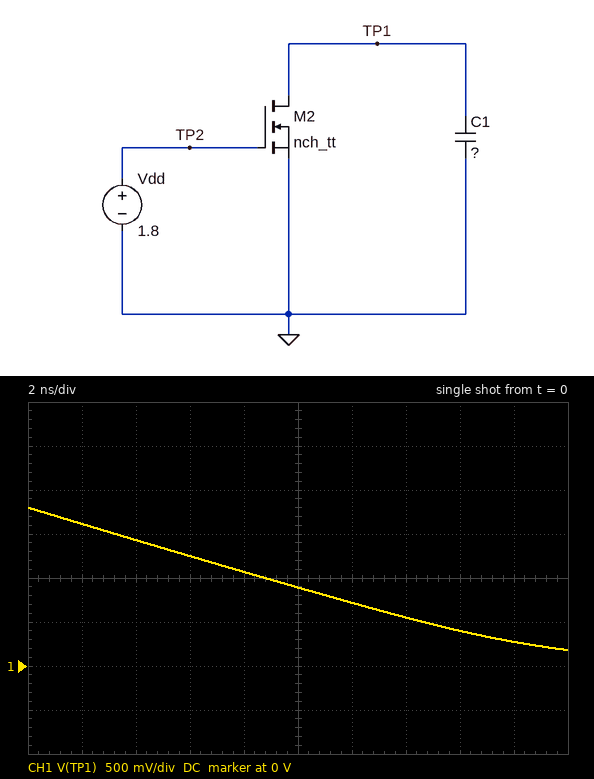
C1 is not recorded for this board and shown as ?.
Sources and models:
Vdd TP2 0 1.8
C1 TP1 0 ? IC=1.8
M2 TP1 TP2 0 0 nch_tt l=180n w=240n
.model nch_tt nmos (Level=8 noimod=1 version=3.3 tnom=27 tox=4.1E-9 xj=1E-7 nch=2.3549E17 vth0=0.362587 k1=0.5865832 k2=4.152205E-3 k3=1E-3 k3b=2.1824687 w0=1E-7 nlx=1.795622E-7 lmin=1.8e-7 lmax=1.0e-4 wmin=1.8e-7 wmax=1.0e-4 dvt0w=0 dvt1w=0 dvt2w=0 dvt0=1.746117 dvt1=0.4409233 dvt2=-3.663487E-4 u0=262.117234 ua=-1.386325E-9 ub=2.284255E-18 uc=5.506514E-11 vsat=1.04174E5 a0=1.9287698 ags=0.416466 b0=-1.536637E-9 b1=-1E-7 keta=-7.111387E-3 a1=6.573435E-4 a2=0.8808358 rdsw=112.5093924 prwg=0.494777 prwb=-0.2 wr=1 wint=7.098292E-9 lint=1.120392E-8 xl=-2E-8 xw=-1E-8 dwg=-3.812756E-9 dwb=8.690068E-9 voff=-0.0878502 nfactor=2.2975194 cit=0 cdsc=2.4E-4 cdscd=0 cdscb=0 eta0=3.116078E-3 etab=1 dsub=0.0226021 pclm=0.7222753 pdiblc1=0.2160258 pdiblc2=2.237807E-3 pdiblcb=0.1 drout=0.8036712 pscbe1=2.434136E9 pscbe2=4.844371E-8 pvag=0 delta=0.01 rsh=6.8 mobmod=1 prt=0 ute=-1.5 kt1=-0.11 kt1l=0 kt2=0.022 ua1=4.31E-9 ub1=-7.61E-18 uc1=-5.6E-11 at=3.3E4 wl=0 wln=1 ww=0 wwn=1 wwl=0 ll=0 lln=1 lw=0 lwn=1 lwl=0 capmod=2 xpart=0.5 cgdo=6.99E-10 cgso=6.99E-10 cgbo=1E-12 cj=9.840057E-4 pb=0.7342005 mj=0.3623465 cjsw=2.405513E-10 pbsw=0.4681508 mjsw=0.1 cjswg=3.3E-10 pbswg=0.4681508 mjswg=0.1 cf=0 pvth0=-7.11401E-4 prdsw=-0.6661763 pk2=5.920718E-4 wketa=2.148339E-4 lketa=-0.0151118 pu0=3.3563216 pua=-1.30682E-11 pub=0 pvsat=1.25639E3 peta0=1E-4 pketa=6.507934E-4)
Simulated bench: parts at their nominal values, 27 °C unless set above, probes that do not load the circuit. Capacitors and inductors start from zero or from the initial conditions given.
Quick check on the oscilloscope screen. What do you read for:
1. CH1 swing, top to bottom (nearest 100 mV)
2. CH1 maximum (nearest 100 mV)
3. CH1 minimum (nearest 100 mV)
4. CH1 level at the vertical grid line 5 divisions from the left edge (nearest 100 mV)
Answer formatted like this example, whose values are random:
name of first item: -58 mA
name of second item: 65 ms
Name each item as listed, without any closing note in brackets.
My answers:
CH1 swing, top to bottom: 1.6 V
CH1 maximum: 1.8 V
CH1 minimum: 200 mV
CH1 level at the vertical grid line 5 divisions from the left edge: 900 mV
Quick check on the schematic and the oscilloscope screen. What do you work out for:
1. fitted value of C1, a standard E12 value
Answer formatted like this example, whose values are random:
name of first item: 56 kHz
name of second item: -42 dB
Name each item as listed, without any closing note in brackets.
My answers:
fitted value of C1, a standard E12 value: 2.2 pF
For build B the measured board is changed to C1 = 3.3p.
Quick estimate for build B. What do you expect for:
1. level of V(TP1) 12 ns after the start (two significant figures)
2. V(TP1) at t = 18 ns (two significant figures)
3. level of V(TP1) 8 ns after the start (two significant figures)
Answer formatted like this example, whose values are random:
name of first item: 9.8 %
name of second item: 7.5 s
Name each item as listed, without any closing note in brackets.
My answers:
level of V(TP1) 12 ns after the start: 1.1 V
V(TP1) at t = 18 ns: 720 mV
level of V(TP1) 8 ns after the start: 1.3 V
